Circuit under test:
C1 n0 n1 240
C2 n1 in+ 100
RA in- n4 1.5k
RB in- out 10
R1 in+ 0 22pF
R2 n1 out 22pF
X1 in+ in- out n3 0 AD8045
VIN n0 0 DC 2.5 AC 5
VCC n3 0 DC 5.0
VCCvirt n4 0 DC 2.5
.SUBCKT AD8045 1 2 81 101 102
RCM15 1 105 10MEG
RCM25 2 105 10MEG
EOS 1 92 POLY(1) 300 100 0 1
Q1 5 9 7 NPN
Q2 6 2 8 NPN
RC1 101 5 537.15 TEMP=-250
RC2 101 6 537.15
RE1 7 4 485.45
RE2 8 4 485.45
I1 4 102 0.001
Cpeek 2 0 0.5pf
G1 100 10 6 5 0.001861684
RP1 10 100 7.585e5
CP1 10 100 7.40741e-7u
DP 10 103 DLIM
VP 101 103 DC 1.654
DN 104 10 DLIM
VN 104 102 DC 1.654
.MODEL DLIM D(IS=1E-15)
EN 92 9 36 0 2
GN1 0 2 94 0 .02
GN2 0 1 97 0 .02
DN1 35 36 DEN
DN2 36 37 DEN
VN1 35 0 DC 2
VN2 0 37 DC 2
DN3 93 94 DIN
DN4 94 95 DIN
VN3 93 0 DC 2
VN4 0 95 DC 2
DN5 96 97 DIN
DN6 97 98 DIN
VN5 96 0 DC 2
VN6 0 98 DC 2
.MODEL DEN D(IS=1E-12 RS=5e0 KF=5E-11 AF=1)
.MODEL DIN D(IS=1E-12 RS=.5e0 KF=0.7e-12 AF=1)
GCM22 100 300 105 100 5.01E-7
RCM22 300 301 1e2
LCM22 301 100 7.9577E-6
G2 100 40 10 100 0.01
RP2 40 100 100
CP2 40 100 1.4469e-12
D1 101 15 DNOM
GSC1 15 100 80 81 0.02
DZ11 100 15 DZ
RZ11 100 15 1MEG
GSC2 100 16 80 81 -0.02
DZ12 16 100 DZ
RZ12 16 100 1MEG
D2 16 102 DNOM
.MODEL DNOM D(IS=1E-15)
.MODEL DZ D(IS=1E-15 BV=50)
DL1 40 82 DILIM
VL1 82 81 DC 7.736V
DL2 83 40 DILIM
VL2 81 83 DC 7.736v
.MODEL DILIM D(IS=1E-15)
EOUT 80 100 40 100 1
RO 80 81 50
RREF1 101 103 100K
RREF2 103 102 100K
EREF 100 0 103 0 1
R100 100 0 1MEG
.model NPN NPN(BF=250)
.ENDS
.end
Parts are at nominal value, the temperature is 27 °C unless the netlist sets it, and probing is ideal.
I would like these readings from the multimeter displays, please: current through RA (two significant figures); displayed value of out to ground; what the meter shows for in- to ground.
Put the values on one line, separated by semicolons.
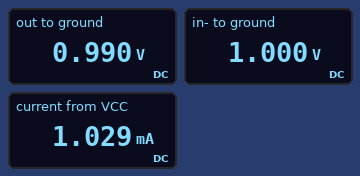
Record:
1.0 mA; 0.990 V; 1.000 V
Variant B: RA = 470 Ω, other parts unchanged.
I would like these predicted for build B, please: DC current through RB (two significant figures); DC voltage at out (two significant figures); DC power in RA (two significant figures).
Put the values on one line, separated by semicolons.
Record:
2.9 mA; 1.1 V; 4.1 mW
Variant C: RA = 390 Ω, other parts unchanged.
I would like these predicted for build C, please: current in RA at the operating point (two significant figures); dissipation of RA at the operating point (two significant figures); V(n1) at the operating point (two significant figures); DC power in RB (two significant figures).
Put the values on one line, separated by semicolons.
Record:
3.5 mA; 4.7 mW; 1.1 V; 120 µW
